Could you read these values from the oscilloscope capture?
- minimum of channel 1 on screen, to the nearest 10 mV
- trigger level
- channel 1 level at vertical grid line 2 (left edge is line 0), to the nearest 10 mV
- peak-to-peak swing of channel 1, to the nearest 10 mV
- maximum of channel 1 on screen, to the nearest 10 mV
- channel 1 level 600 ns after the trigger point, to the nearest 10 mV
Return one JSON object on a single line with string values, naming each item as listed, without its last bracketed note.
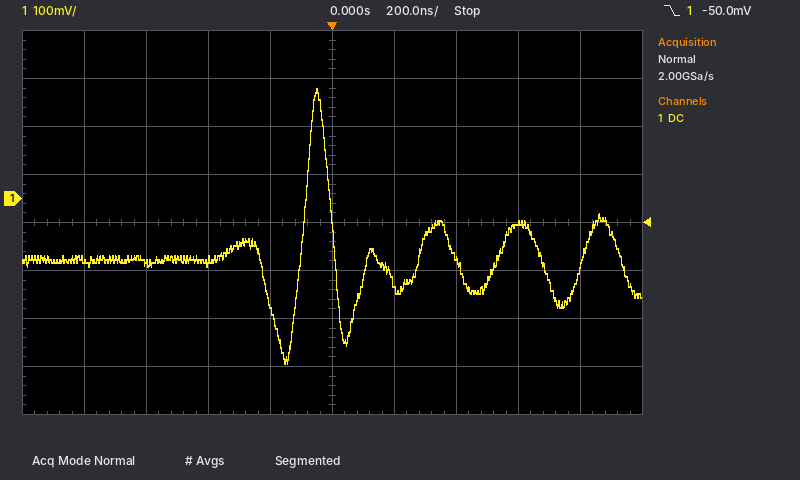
{"minimum of channel 1 on screen, to the nearest 10 mV": "-340 mV", "trigger level": "-50.0 mV", "channel 1 level at vertical grid line 2 (left edge is line 0), to the nearest 10 mV": "-130 mV", "peak-to-peak swing of channel 1, to the nearest 10 mV": "570 mV", "maximum of channel 1 on screen, to the nearest 10 mV": "230 mV", "channel 1 level 600 ns after the trigger point, to the nearest 10 mV": "-50 mV"}
